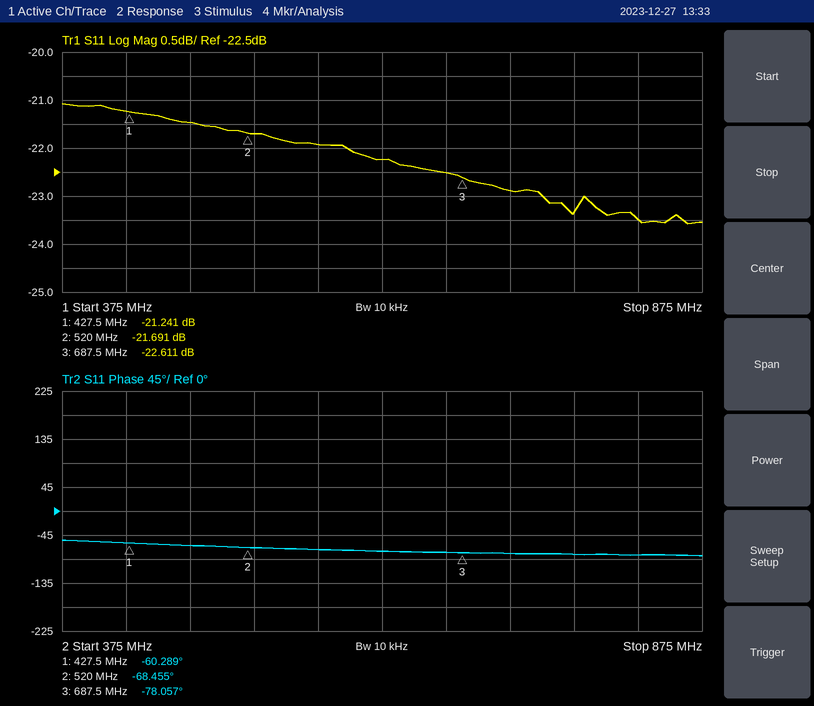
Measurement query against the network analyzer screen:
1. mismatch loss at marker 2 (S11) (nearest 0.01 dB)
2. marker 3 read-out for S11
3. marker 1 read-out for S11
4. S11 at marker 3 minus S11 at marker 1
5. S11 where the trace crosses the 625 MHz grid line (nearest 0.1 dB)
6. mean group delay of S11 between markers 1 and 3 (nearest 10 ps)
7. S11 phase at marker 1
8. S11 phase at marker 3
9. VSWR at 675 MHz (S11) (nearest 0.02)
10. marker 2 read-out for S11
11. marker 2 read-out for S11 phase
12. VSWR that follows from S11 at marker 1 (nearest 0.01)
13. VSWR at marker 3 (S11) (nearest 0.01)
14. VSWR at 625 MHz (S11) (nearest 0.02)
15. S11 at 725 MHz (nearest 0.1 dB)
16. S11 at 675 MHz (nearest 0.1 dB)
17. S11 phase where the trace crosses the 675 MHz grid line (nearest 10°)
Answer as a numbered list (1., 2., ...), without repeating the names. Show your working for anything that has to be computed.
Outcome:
1. −10 log10(1 − 10^(-21.691/10)) ≈ 0.03 dB
2. -22.611 dB
3. -21.241 dB
4. -22.611 − (-21.241) = -1.370 dB
5. -22.2 dB
6. −(-78.057° − (-60.289°))/(360° × 260 MHz) ≈ 190 ps
7. -60.289°
8. -78.057°
9. |Γ| = 10^(-22.5/20) = 0.0750; VSWR = (1 + 0.0750)/(1 − 0.0750) ≈ 1.16
10. -21.691 dB
11. -68.455°
12. (1 + 0.0867)/(1 − 0.0867) ≈ 1.19
13. (1 + 0.0740)/(1 − 0.0740) ≈ 1.16
14. |Γ| = 10^(-22.2/20) = 0.0776; VSWR = (1 + 0.0776)/(1 − 0.0776) ≈ 1.17, so 1.16 to the nearest 0.02
15. -22.9 dB
16. -22.5 dB
17. -80°
